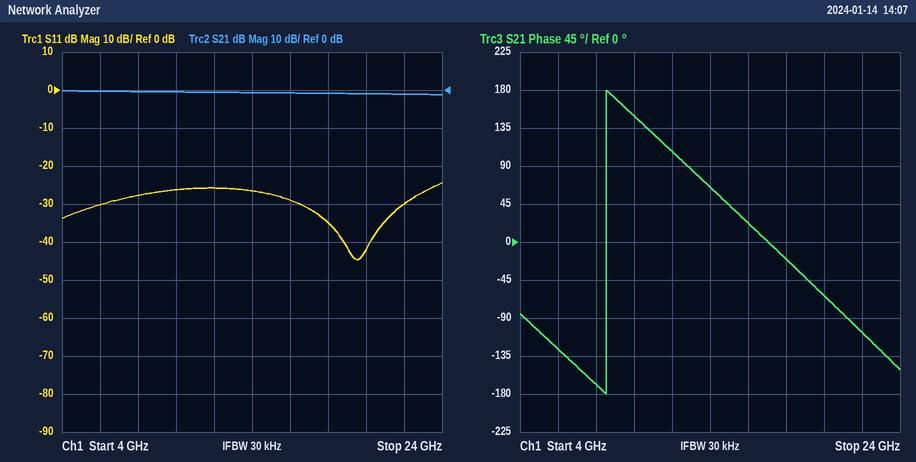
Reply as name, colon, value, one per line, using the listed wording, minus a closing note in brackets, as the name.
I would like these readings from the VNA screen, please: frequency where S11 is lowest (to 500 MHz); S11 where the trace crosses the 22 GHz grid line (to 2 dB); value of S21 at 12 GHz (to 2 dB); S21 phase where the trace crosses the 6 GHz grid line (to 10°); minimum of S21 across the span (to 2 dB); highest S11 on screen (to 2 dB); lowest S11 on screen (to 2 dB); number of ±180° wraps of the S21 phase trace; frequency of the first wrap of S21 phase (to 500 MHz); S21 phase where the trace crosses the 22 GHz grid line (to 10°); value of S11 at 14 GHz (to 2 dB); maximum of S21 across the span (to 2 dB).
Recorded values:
frequency where S11 is lowest: 19.5 GHz
S11 where the trace crosses the 22 GHz grid line: -30 dB
value of S21 at 12 GHz: 0 dB
S21 phase where the trace crosses the 6 GHz grid line: -130°
minimum of S21 across the span: -2 dB
highest S11 on screen: -24 dB
lowest S11 on screen: -44 dB
number of ±180° wraps of the S21 phase trace: 1
frequency of the first wrap of S21 phase: 8.5 GHz
S21 phase where the trace crosses the 22 GHz grid line: -110°
value of S11 at 14 GHz: -26 dB
maximum of S21 across the span: 0 dB
